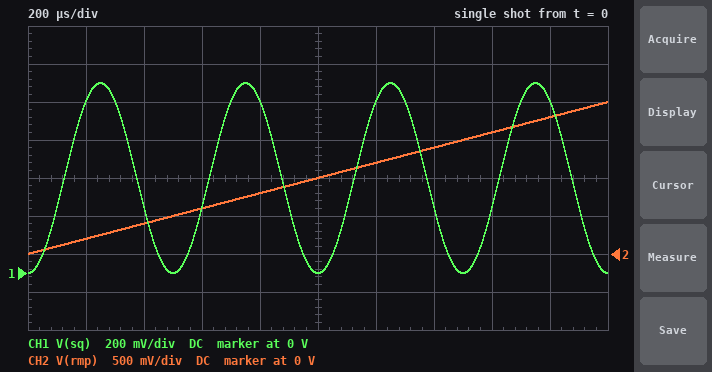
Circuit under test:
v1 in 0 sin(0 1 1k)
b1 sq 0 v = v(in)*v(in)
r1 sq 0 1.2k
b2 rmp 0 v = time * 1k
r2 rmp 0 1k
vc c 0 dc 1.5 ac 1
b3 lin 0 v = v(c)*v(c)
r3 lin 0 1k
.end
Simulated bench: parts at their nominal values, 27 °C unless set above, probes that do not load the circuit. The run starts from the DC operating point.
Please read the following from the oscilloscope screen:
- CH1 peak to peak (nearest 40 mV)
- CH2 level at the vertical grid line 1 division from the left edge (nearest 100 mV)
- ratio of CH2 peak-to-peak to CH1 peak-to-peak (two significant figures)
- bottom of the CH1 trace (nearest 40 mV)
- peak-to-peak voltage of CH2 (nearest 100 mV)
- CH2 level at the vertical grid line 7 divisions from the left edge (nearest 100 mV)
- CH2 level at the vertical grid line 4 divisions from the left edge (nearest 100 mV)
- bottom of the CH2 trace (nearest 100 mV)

1.00 V
200 mV
2.0
0 V
2.0 V
1.4 V
800 mV
0 V
